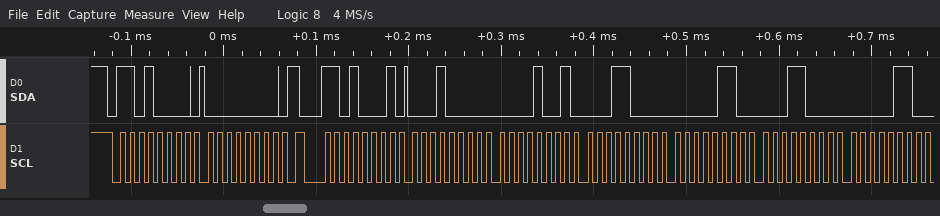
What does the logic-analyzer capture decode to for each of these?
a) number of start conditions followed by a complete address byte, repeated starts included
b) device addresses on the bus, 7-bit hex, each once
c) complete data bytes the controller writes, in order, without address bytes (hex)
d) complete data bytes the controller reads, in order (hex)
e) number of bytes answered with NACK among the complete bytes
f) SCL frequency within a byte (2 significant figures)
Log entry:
2
0x68
00
10 09 18 06 18 06
0
100 kHz
